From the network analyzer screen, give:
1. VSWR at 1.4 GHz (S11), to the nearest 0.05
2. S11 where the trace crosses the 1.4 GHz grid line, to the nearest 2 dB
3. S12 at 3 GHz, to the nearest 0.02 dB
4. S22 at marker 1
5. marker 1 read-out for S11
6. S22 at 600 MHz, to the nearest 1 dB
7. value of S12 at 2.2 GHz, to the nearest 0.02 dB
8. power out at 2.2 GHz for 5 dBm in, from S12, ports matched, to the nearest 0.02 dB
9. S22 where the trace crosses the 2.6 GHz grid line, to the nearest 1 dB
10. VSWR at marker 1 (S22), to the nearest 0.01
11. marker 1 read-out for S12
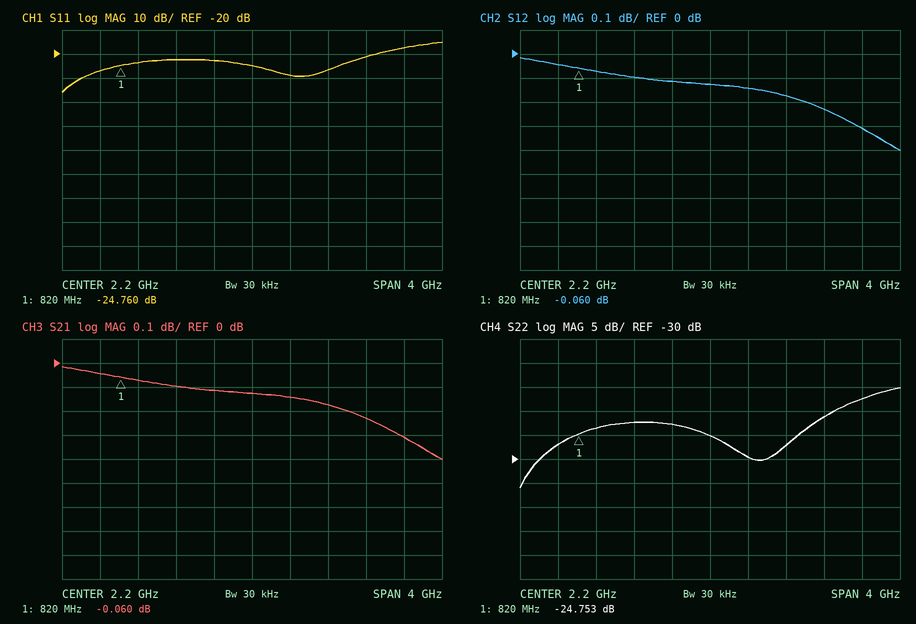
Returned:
1.15
-22 dB
-0.18 dB
-24.753 dB
-24.760 dB
-27 dB
-0.12 dB
4.88 dBm
-30 dB
1.12
-0.060 dB
